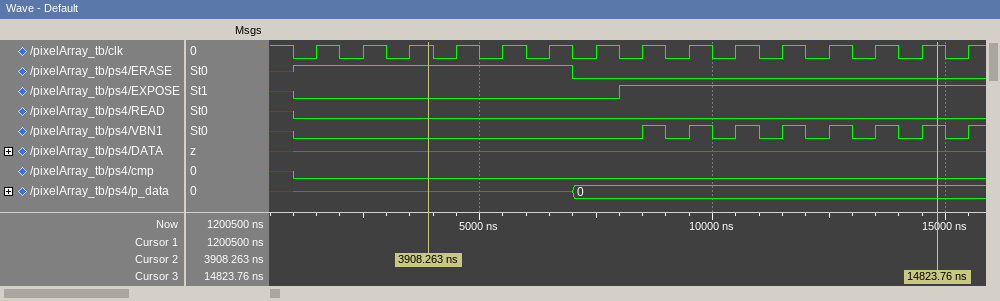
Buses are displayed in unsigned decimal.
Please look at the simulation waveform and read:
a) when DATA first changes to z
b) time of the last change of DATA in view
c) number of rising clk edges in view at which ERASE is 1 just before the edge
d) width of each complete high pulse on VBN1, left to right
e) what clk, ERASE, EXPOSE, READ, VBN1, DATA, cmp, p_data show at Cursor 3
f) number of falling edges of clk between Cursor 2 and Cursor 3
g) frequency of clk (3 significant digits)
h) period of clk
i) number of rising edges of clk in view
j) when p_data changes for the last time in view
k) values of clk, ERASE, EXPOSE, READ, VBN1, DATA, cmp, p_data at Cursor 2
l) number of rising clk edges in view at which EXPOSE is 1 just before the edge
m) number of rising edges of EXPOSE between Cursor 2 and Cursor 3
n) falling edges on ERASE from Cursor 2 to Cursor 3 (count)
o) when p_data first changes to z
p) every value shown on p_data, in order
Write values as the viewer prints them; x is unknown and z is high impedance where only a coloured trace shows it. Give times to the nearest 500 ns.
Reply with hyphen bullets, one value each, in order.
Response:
- 1000 ns
- 1000 ns
- 6
- 500 ns, 500 ns, 500 ns, 500 ns, 500 ns, 500 ns, 500 ns
- clk=1, ERASE=0, EXPOSE=1, READ=0, VBN1=1, DATA=z, cmp=0, p_data=0
- 11
- 1.00 MHz
- 1000 ns
- 15
- 7000 ns
- clk=1, ERASE=1, EXPOSE=0, READ=0, VBN1=0, DATA=z, cmp=0, p_data=z
- 8
- 1
- 1
- 1000 ns
- x, z, 0
